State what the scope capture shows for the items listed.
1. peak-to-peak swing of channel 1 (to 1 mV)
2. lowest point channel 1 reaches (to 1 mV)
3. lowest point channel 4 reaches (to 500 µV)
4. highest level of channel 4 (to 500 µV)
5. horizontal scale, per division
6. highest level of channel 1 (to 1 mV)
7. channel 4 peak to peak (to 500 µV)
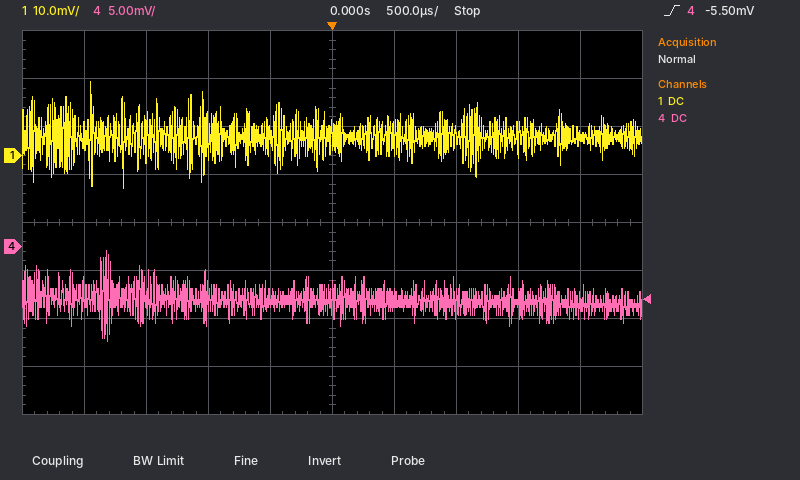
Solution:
22 mV
-7 mV
-10.0 mV
-500 µV
500 µs
15 mV
9.5 mV
